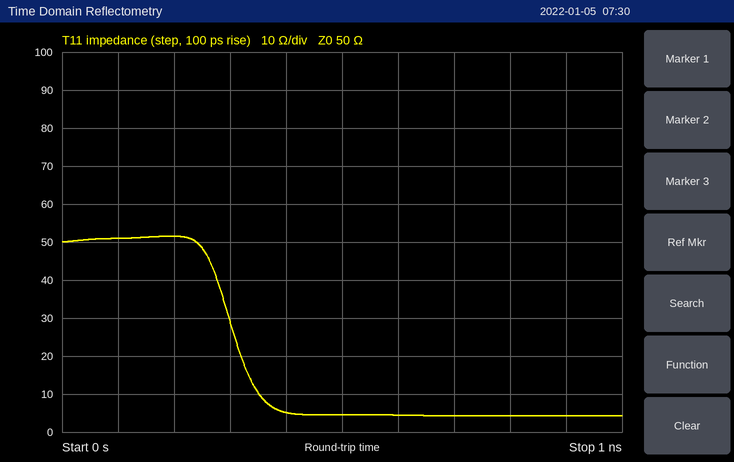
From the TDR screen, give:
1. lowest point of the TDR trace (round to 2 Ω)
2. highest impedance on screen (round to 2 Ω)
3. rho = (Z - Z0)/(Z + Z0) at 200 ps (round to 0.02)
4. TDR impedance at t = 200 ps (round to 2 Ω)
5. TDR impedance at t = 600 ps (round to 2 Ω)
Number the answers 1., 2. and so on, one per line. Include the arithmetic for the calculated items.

1. 4 Ω
2. 52 Ω
3. (52 − 50)/(52 + 50) ≈ +0.02
4. 52 Ω
5. 4 Ω
